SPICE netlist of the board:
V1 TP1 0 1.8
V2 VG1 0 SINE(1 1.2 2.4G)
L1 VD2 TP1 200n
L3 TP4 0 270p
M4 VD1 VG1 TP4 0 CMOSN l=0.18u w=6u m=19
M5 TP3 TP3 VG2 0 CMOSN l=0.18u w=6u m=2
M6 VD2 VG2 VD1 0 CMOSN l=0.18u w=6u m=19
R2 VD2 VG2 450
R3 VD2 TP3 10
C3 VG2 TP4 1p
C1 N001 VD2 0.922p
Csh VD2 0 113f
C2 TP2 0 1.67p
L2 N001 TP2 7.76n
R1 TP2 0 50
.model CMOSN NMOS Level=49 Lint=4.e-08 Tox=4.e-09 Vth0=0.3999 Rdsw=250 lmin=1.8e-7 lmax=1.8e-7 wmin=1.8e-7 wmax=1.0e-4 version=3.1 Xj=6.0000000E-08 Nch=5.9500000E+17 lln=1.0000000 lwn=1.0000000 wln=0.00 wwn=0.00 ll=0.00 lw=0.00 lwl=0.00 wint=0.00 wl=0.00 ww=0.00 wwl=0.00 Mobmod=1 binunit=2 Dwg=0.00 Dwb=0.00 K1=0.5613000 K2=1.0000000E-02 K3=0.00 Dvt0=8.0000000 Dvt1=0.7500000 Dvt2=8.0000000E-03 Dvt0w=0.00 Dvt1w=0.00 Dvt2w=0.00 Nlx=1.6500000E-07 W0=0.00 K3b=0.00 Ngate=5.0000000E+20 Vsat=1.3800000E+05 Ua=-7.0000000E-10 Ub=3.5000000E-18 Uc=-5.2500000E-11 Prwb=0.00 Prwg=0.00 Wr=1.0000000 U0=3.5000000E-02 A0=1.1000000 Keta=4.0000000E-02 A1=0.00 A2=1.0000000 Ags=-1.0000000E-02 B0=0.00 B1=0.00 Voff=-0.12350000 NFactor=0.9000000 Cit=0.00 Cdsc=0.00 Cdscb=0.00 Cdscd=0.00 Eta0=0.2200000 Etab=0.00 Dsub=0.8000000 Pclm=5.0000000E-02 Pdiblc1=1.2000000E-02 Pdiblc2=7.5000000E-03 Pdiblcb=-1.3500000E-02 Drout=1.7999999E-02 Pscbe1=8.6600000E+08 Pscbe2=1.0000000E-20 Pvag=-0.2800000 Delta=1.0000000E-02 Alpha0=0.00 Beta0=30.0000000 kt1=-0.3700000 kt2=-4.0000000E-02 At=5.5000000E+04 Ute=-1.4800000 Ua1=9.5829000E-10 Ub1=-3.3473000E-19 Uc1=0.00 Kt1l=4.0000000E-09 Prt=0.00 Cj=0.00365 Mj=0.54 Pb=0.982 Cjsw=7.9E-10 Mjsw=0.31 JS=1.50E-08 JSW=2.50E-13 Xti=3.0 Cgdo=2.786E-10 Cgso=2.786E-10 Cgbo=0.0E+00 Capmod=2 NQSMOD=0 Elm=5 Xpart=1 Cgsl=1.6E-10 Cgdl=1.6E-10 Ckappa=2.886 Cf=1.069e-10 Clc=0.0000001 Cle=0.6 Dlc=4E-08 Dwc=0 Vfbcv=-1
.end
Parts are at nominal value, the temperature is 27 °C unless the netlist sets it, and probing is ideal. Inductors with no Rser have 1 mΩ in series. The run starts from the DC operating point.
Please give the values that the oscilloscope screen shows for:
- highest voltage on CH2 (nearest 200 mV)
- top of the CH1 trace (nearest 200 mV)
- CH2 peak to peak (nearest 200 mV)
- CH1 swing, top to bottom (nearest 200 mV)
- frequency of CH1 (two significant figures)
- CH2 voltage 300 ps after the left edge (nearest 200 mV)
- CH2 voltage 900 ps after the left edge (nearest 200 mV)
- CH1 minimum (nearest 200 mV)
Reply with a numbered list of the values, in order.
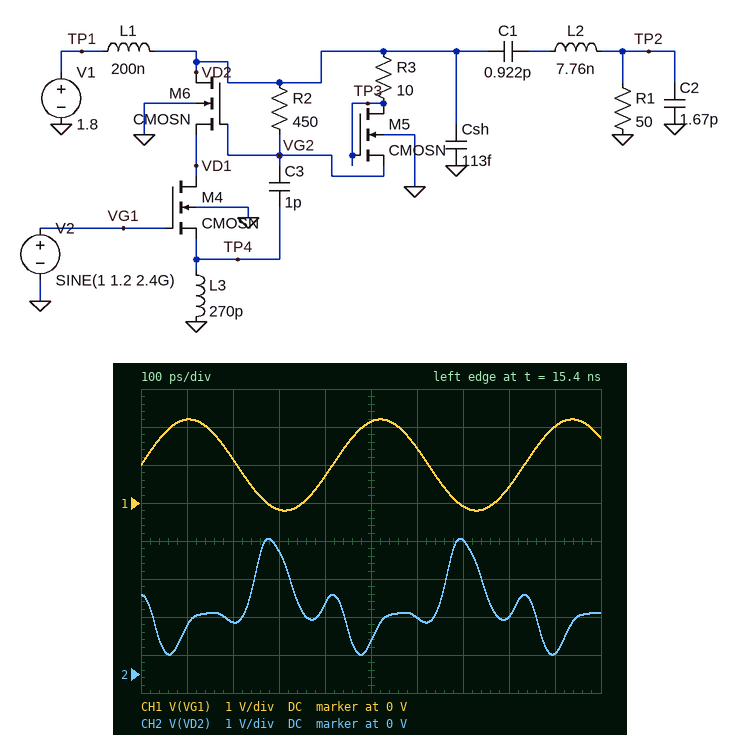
1. 3.6 V
2. 2.2 V
3. 3.0 V
4. 2.4 V
5. 2.4 GHz
6. 3.2 V
7. 600 mV
8. -200 mV
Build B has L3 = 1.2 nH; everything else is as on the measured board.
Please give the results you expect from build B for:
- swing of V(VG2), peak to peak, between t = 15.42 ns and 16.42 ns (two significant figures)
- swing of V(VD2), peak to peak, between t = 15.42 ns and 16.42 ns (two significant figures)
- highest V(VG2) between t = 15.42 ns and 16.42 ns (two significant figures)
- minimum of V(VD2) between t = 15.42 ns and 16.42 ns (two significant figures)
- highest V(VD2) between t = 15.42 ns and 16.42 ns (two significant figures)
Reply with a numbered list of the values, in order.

1. 1.2 V
2. 2.2 V
3. 2.5 V
4. 840 mV
5. 3.0 V
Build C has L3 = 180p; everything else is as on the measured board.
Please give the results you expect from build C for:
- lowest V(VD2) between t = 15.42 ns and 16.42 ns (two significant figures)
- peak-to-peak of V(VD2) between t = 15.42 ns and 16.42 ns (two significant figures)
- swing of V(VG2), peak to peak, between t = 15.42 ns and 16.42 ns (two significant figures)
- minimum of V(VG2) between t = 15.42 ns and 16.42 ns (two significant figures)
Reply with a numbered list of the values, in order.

1. 520 mV
2. 3.0 V
3. 600 mV
4. 1.7 V
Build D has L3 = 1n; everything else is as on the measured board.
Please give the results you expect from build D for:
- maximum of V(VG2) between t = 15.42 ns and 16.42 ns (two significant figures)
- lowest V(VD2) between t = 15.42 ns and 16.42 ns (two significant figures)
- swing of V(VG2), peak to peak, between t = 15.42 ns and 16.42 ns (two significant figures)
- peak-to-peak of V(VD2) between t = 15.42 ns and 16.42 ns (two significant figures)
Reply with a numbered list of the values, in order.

1. 2.4 V
2. 720 mV
3. 1.2 V
4. 2.5 V
